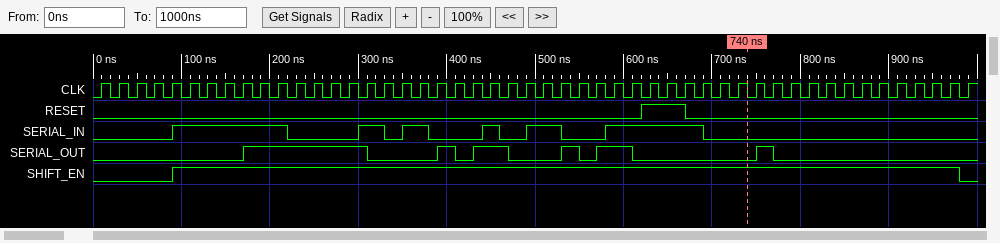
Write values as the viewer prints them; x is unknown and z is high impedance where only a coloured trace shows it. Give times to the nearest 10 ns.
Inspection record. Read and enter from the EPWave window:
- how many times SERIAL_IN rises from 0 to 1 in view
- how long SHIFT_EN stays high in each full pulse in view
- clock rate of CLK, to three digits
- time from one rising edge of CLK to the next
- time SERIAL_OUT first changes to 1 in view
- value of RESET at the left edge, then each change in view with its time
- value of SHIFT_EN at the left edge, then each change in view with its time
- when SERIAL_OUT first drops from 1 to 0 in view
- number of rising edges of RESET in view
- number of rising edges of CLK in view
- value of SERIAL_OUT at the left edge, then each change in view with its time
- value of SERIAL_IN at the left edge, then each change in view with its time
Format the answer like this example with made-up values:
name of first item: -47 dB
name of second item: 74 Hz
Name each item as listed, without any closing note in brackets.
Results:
how many times SERIAL_IN rises from 0 to 1 in view: 6
how long SHIFT_EN stays high in each full pulse in view: 890 ns
clock rate of CLK, to three digits: 50.0 MHz
time from one rising edge of CLK to the next: 20 ns
time SERIAL_OUT first changes to 1 in view: 170 ns
value of RESET at the left edge, then each change in view with its time: 0, 1 at 620 ns, 0 at 670 ns
value of SHIFT_EN at the left edge, then each change in view with its time: 0, 1 at 90 ns, 0 at 980 ns
when SERIAL_OUT first drops from 1 to 0 in view: 310 ns
number of rising edges of RESET in view: 1
number of rising edges of CLK in view: 50
value of SERIAL_OUT at the left edge, then each change in view with its time: 0, 1 at 170 ns, 0 at 310 ns, 1 at 390 ns, 0 at 410 ns, 1 at 430 ns, 0 at 470 ns, 1 at 530 ns, 0 at 550 ns, 1 at 570 ns, 0 at 610 ns, 1 at 750 ns, 0 at 770 ns
value of SERIAL_IN at the left edge, then each change in view with its time: 0, 1 at 90 ns, 0 at 220 ns, 1 at 300 ns, 0 at 330 ns, 1 at 350 ns, 0 at 380 ns, 1 at 440 ns, 0 at 460 ns, 1 at 490 ns, 0 at 530 ns, 1 at 580 ns, 0 at 690 ns
